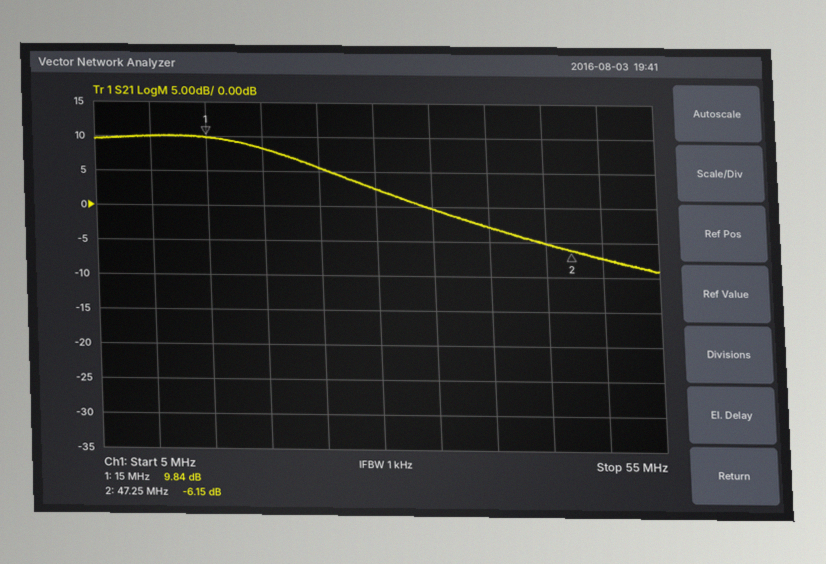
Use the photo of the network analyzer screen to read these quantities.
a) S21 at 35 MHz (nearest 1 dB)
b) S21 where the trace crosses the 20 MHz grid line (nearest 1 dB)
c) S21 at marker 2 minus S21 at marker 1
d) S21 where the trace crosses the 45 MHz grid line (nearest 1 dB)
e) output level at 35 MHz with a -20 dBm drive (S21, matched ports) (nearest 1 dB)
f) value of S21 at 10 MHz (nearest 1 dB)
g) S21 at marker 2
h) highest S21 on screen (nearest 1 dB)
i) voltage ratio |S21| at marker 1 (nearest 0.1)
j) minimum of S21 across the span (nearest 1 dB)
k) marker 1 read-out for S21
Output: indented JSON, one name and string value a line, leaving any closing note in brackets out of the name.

{
  "S21 at 35 MHz": "0 dB",
  "S21 where the trace crosses the 20 MHz grid line": "8 dB",
  "S21 at marker 2 minus S21 at marker 1": "-15.99 dB",
  "S21 where the trace crosses the 45 MHz grid line": "-5 dB",
  "output level at 35 MHz with a -20 dBm drive (S21, matched ports)": "-20 dBm",
  "value of S21 at 10 MHz": "10 dB",
  "S21 at marker 2": "-6.15 dB",
  "highest S21 on screen": "10 dB",
  "voltage ratio |S21| at marker 1": "3.1",
  "minimum of S21 across the span": "-9 dB",
  "marker 1 read-out for S21": "9.84 dB"
}
